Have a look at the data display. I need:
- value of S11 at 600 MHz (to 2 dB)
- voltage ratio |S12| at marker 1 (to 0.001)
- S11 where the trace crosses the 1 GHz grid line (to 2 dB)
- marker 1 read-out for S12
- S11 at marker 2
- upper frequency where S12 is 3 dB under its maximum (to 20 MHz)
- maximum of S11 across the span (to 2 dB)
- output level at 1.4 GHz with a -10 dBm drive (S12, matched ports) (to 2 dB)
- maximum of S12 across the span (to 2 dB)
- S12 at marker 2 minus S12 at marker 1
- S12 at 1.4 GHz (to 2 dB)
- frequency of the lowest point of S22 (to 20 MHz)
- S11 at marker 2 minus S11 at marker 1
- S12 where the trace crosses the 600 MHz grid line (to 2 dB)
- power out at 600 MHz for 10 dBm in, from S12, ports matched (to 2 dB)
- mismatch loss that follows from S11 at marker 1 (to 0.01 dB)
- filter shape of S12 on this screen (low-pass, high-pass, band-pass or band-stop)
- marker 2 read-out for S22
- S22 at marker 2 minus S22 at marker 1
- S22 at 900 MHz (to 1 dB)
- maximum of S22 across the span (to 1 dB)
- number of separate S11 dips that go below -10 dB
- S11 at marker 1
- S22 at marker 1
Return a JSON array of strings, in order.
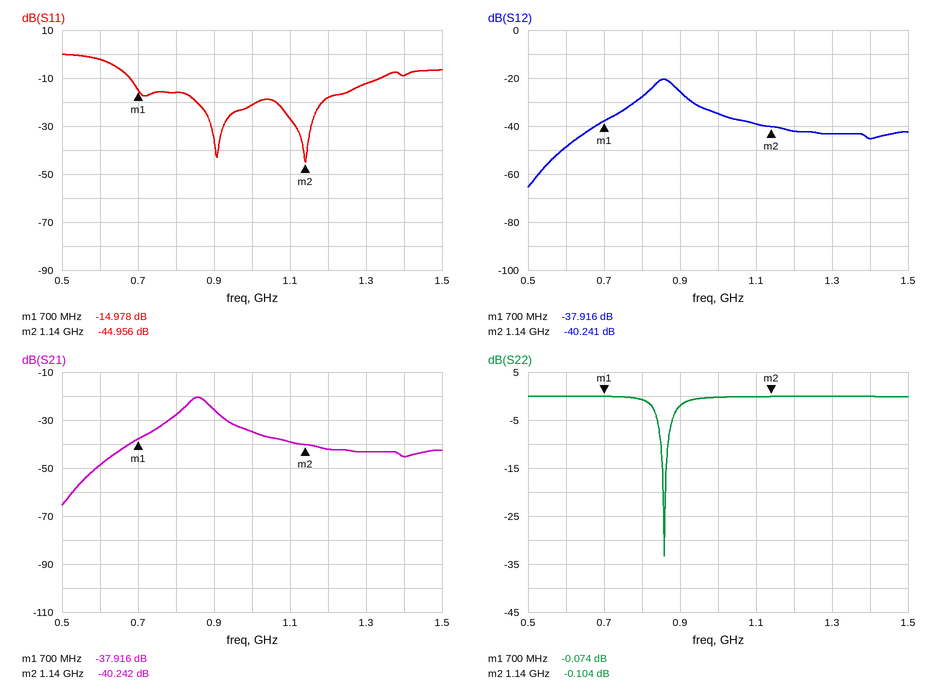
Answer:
["-2 dB", "0.013", "-22 dB", "-37.916 dB", "-44.956 dB", "880 MHz", "0 dB", "-56 dBm", "-20 dB", "-2.325 dB", "-46 dB", "860 MHz", "-29.978 dB", "-48 dB", "-38 dBm", "0.14 dB", "band-pass", "-0.104 dB", "-0.030 dB", "-2 dB", "0 dB", "2", "-14.978 dB", "-0.074 dB"]
